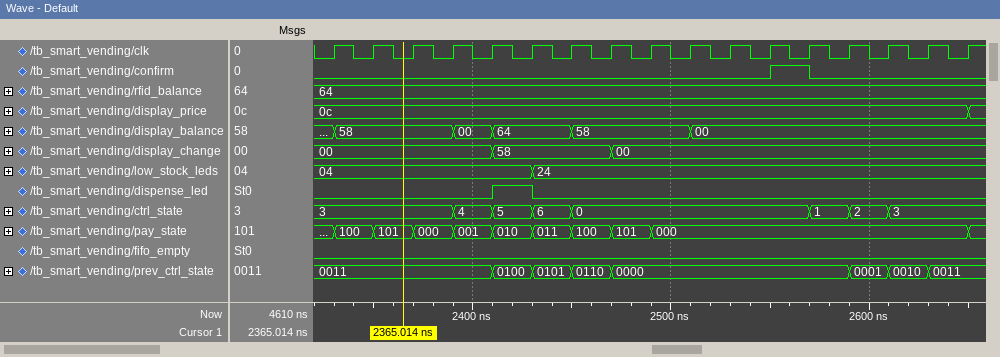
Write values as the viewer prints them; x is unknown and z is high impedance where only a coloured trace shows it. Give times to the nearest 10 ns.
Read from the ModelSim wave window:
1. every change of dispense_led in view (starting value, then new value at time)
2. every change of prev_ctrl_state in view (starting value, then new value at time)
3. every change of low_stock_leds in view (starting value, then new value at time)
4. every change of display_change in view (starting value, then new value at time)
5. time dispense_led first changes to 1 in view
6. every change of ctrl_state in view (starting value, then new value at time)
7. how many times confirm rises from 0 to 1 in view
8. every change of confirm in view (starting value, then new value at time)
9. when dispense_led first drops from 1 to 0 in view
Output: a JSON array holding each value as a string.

["0, 1 at 2410 ns, 0 at 2430 ns", "0011, 0100 at 2410 ns, 0101 at 2430 ns, 0110 at 2450 ns, 0000 at 2470 ns, 0001 at 2590 ns, 0010 at 2610 ns, 0011 at 2630 ns", "04, 24 at 2430 ns", "00, 58 at 2410 ns, 00 at 2470 ns", "2410 ns", "3, 4 at 2390 ns, 5 at 2410 ns, 6 at 2430 ns, 0 at 2450 ns, 1 at 2570 ns, 2 at 2590 ns, 3 at 2610 ns", "1", "0, 1 at 2550 ns, 0 at 2570 ns", "2430 ns"]
